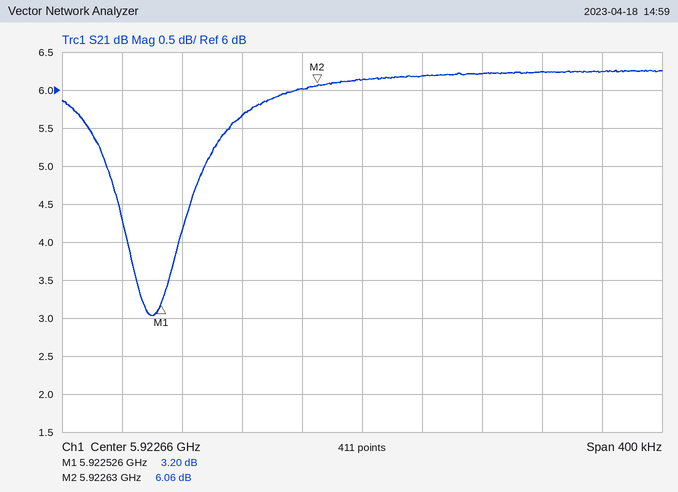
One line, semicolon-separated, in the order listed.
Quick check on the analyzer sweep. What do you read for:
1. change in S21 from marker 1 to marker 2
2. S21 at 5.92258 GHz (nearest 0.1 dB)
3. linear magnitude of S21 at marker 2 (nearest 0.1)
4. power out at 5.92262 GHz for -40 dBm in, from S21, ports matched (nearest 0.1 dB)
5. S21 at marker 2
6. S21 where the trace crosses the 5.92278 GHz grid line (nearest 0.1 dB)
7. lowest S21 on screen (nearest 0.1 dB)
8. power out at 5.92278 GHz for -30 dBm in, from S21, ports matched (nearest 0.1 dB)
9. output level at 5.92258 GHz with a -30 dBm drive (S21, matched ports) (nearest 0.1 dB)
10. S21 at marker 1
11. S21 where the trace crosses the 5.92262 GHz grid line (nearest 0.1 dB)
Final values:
2.86 dB; 5.7 dB; 2.0; -34.0 dBm; 6.06 dB; 6.2 dB; 3.0 dB; -23.8 dBm; -24.3 dBm; 3.20 dB; 6.0 dB
